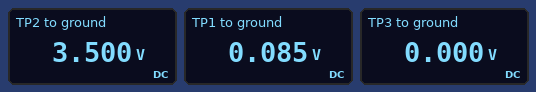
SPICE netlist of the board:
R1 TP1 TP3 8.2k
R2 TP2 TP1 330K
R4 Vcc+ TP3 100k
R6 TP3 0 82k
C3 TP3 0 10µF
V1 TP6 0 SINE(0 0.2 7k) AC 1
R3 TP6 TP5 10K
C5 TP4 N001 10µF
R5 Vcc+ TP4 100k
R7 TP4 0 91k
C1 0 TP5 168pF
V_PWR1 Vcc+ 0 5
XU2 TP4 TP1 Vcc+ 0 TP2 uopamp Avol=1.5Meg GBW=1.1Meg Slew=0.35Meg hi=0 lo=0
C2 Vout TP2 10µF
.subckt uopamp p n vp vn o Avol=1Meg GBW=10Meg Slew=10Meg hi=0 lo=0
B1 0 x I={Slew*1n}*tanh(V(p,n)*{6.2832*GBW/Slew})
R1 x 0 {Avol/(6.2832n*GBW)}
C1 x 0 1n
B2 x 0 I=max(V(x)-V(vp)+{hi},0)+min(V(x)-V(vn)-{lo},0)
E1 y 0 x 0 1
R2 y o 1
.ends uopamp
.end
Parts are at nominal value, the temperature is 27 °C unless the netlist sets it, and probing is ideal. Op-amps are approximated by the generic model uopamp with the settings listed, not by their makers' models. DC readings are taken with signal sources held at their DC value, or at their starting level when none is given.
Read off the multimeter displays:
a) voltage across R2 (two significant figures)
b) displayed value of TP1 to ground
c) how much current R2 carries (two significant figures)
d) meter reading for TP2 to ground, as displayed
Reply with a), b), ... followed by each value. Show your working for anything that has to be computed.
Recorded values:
a) 3.5 V - 85 mV = 3.4 V
b) 0.085 V
c) (3.5 V - 85 mV) / 330 kΩ = 10 µA
d) 3.500 V
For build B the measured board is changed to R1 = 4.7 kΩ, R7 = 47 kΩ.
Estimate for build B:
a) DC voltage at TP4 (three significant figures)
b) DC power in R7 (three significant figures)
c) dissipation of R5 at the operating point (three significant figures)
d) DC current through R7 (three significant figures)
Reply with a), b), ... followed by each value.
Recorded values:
a) 1.60 V
b) 54.4 µW
c) 116 µW
d) 34.0 µA
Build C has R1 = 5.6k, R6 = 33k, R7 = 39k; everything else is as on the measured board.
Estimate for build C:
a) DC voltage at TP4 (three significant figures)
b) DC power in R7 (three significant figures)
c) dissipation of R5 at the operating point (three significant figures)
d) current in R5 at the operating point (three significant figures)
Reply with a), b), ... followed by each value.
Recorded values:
a) 1.40 V
b) 50.5 µW
c) 129 µW
d) 36.0 µA
